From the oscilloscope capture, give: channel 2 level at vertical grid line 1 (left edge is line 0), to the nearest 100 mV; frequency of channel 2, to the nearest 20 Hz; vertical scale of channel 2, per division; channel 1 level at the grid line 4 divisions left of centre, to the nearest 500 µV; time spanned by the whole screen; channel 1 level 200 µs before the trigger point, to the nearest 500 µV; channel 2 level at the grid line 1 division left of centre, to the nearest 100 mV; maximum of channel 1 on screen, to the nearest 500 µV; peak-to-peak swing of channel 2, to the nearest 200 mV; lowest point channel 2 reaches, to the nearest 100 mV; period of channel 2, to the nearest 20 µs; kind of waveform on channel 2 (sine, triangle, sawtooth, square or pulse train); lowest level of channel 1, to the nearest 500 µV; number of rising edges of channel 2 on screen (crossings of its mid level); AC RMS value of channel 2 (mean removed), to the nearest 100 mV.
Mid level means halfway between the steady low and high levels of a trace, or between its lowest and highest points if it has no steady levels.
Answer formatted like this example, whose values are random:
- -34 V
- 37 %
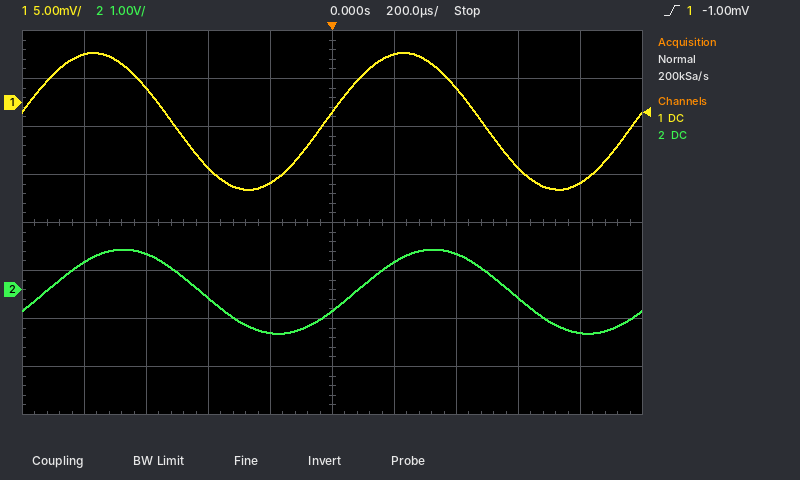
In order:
- 600 mV
- 1.00 kHz
- 1 V
- 5.0 mV
- 2 ms
- -8.5 mV
- -900 mV
- 5.0 mV
- 1.8 V
- -900 mV
- 1.00 ms
- sine
- -9.0 mV
- 2
- 600 mV
